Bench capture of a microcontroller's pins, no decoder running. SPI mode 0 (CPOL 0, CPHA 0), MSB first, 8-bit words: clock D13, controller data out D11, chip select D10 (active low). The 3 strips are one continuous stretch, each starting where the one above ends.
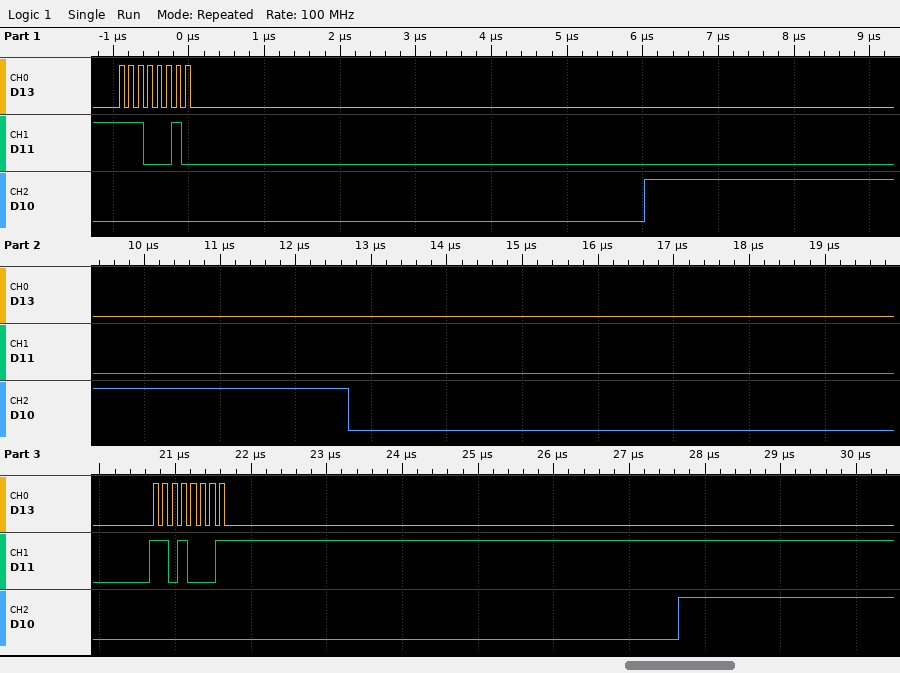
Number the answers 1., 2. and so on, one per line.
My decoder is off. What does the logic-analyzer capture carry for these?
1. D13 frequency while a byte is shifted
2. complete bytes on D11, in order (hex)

1. 8 MHz
2. E2 D1
